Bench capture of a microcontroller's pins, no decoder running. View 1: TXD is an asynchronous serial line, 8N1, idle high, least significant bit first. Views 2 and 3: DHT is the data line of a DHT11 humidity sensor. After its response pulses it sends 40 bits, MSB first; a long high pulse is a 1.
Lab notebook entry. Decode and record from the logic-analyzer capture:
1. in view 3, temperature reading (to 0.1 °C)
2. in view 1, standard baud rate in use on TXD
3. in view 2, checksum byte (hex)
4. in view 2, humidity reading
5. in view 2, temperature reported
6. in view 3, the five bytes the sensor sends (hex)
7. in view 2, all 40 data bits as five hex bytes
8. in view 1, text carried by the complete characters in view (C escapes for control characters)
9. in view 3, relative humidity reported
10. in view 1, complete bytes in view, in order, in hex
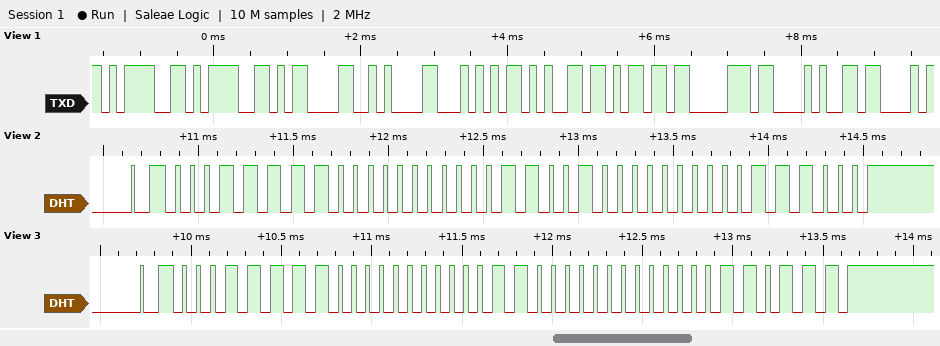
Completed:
24.0 °C
9600 baud
0x38
31 %
25.0 °C
1F 00 18 00 37
1F 00 19 00 38
"==\r\nTemp(C"
31 %
0x3D 0x3D 0x0D 0x0A 0x54 0x65 0x6D 0x70 0x28 0x43
